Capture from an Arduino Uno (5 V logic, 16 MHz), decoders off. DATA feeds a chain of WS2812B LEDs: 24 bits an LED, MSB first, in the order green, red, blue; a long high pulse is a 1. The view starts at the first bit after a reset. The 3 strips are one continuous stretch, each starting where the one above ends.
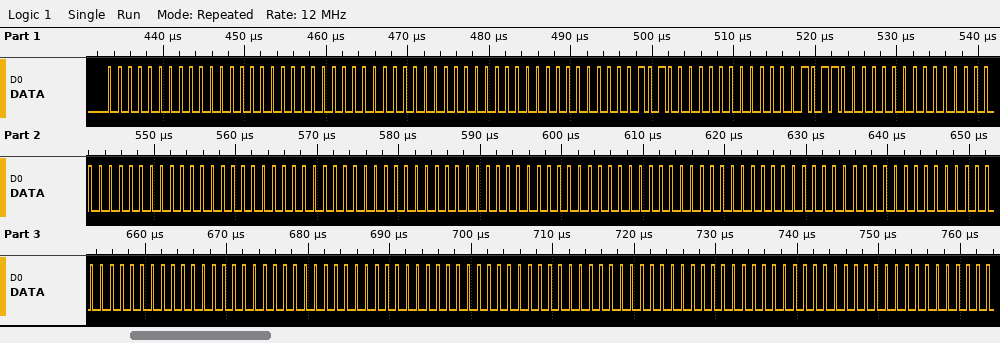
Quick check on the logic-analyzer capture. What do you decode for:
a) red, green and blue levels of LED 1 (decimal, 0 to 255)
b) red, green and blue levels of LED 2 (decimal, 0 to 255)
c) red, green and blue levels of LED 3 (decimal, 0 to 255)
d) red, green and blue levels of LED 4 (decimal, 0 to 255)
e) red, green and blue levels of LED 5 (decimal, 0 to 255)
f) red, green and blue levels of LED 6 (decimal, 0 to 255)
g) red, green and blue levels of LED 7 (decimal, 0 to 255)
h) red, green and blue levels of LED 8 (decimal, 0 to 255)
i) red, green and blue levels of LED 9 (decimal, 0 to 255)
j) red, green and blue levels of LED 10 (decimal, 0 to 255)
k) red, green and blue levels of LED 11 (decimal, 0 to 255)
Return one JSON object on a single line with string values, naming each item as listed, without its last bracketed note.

{"red, green and blue levels of LED 1": "0, 0, 0", "red, green and blue levels of LED 2": "0, 0, 0", "red, green and blue levels of LED 3": "0, 10, 11", "red, green and blue levels of LED 4": "0, 0, 0", "red, green and blue levels of LED 5": "0, 0, 0", "red, green and blue levels of LED 6": "0, 0, 0", "red, green and blue levels of LED 7": "0, 0, 0", "red, green and blue levels of LED 8": "0, 0, 0", "red, green and blue levels of LED 9": "0, 0, 0", "red, green and blue levels of LED 10": "0, 0, 0", "red, green and blue levels of LED 11": "0, 0, 0"}
